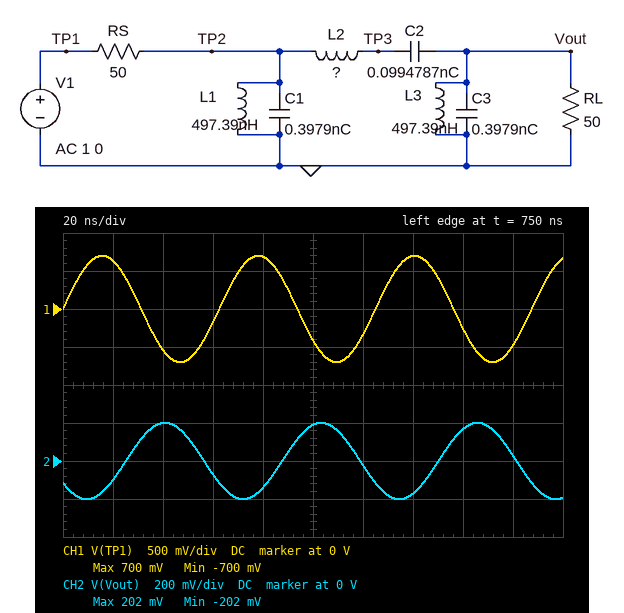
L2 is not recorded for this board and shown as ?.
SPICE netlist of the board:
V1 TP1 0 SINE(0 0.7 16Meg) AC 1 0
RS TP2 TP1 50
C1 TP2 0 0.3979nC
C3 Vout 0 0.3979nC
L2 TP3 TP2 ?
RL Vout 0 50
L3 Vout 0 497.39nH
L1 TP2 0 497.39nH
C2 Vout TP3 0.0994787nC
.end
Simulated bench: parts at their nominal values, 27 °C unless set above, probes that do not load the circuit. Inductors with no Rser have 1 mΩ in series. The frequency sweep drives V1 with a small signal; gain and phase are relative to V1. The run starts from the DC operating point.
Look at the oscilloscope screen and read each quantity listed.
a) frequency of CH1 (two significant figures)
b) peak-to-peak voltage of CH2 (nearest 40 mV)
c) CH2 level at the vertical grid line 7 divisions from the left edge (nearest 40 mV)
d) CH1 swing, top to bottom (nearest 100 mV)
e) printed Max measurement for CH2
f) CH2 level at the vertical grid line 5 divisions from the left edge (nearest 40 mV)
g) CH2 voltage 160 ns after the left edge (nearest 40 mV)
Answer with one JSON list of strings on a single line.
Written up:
["16 MHz", "400 mV", "-160 mV", "1.4 V", "202 mV", "200 mV", "160 mV"]
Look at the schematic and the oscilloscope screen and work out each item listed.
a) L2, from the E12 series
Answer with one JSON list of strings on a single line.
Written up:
["2.2 µH"]
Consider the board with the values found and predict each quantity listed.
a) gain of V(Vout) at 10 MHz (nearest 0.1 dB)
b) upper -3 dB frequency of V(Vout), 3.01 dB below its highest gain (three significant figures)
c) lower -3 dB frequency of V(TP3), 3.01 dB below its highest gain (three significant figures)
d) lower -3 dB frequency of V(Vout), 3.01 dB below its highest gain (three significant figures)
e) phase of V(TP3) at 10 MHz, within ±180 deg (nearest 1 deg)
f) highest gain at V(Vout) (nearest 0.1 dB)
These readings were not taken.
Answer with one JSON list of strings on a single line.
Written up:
["-6.1 dB", "15.3 MHz", "7.19 MHz", "7.82 MHz", "-60 deg", "-6.0 dB"]
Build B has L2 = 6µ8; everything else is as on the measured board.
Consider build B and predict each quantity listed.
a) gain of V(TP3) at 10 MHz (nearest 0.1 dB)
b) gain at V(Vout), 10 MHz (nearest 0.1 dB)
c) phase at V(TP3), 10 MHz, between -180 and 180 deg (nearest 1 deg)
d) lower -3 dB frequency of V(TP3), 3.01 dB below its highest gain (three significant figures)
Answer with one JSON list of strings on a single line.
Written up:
["-6.8 dB", "-16.9 dB", "-127 deg", "5.49 MHz"]
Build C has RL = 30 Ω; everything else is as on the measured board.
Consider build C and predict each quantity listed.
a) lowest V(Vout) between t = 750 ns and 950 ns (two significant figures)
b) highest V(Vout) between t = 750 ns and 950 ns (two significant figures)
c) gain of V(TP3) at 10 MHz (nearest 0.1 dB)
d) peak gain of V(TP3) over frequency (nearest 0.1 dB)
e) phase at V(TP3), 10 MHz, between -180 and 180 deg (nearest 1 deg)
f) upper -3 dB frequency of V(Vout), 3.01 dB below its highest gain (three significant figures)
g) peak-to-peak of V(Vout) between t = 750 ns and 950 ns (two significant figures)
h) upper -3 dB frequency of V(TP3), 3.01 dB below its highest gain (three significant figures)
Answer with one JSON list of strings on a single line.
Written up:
["-130 mV", "130 mV", "6.1 dB", "6.9 dB", "-60 deg", "14.7 MHz", "270 mV", "13.0 MHz"]
